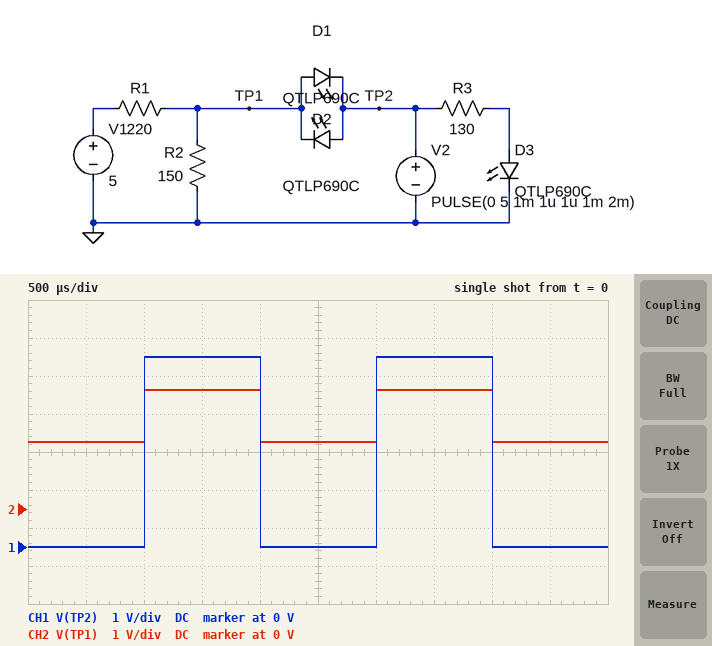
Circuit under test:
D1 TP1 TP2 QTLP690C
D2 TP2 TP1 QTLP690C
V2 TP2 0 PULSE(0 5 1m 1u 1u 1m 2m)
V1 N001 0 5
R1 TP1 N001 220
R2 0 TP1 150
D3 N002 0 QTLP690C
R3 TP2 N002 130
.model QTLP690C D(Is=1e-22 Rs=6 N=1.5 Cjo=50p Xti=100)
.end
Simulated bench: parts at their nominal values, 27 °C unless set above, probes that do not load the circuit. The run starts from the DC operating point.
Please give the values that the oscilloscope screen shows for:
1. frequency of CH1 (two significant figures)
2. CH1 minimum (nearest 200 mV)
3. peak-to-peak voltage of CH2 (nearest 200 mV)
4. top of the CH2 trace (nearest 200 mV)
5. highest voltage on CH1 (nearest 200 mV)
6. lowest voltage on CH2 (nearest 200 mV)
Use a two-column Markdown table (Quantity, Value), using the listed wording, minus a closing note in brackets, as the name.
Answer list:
| Quantity | Value |
|---|---|
| frequency of CH1 | 500 Hz |
| CH1 minimum | 0 V |
| peak-to-peak voltage of CH2 | 1.4 V |
| top of the CH2 trace | 3.2 V |
| highest voltage on CH1 | 5.0 V |
| lowest voltage on CH2 | 1.8 V |
